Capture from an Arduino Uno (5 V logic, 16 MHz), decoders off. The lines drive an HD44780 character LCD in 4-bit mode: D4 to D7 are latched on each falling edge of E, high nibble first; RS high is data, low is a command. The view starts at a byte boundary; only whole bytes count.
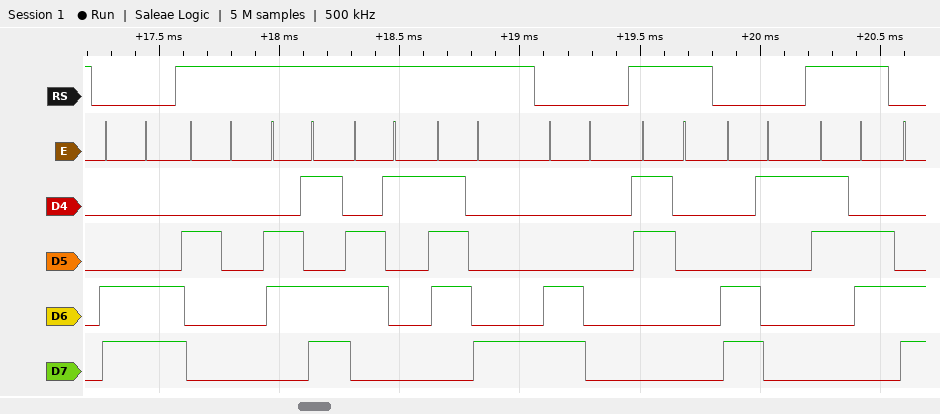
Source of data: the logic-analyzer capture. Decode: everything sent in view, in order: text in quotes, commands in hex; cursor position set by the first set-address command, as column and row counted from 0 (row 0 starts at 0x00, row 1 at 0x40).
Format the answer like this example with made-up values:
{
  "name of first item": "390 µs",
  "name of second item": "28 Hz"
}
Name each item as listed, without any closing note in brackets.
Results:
{
  "everything sent in view, in order: text in quotes, commands in hex": "0xCC \" max\" 0xC0 \"0\" 0xC1 \"6\"",
  "cursor position set by the first set-address command, as column and row counted from 0": "column 12, row 1"
}
